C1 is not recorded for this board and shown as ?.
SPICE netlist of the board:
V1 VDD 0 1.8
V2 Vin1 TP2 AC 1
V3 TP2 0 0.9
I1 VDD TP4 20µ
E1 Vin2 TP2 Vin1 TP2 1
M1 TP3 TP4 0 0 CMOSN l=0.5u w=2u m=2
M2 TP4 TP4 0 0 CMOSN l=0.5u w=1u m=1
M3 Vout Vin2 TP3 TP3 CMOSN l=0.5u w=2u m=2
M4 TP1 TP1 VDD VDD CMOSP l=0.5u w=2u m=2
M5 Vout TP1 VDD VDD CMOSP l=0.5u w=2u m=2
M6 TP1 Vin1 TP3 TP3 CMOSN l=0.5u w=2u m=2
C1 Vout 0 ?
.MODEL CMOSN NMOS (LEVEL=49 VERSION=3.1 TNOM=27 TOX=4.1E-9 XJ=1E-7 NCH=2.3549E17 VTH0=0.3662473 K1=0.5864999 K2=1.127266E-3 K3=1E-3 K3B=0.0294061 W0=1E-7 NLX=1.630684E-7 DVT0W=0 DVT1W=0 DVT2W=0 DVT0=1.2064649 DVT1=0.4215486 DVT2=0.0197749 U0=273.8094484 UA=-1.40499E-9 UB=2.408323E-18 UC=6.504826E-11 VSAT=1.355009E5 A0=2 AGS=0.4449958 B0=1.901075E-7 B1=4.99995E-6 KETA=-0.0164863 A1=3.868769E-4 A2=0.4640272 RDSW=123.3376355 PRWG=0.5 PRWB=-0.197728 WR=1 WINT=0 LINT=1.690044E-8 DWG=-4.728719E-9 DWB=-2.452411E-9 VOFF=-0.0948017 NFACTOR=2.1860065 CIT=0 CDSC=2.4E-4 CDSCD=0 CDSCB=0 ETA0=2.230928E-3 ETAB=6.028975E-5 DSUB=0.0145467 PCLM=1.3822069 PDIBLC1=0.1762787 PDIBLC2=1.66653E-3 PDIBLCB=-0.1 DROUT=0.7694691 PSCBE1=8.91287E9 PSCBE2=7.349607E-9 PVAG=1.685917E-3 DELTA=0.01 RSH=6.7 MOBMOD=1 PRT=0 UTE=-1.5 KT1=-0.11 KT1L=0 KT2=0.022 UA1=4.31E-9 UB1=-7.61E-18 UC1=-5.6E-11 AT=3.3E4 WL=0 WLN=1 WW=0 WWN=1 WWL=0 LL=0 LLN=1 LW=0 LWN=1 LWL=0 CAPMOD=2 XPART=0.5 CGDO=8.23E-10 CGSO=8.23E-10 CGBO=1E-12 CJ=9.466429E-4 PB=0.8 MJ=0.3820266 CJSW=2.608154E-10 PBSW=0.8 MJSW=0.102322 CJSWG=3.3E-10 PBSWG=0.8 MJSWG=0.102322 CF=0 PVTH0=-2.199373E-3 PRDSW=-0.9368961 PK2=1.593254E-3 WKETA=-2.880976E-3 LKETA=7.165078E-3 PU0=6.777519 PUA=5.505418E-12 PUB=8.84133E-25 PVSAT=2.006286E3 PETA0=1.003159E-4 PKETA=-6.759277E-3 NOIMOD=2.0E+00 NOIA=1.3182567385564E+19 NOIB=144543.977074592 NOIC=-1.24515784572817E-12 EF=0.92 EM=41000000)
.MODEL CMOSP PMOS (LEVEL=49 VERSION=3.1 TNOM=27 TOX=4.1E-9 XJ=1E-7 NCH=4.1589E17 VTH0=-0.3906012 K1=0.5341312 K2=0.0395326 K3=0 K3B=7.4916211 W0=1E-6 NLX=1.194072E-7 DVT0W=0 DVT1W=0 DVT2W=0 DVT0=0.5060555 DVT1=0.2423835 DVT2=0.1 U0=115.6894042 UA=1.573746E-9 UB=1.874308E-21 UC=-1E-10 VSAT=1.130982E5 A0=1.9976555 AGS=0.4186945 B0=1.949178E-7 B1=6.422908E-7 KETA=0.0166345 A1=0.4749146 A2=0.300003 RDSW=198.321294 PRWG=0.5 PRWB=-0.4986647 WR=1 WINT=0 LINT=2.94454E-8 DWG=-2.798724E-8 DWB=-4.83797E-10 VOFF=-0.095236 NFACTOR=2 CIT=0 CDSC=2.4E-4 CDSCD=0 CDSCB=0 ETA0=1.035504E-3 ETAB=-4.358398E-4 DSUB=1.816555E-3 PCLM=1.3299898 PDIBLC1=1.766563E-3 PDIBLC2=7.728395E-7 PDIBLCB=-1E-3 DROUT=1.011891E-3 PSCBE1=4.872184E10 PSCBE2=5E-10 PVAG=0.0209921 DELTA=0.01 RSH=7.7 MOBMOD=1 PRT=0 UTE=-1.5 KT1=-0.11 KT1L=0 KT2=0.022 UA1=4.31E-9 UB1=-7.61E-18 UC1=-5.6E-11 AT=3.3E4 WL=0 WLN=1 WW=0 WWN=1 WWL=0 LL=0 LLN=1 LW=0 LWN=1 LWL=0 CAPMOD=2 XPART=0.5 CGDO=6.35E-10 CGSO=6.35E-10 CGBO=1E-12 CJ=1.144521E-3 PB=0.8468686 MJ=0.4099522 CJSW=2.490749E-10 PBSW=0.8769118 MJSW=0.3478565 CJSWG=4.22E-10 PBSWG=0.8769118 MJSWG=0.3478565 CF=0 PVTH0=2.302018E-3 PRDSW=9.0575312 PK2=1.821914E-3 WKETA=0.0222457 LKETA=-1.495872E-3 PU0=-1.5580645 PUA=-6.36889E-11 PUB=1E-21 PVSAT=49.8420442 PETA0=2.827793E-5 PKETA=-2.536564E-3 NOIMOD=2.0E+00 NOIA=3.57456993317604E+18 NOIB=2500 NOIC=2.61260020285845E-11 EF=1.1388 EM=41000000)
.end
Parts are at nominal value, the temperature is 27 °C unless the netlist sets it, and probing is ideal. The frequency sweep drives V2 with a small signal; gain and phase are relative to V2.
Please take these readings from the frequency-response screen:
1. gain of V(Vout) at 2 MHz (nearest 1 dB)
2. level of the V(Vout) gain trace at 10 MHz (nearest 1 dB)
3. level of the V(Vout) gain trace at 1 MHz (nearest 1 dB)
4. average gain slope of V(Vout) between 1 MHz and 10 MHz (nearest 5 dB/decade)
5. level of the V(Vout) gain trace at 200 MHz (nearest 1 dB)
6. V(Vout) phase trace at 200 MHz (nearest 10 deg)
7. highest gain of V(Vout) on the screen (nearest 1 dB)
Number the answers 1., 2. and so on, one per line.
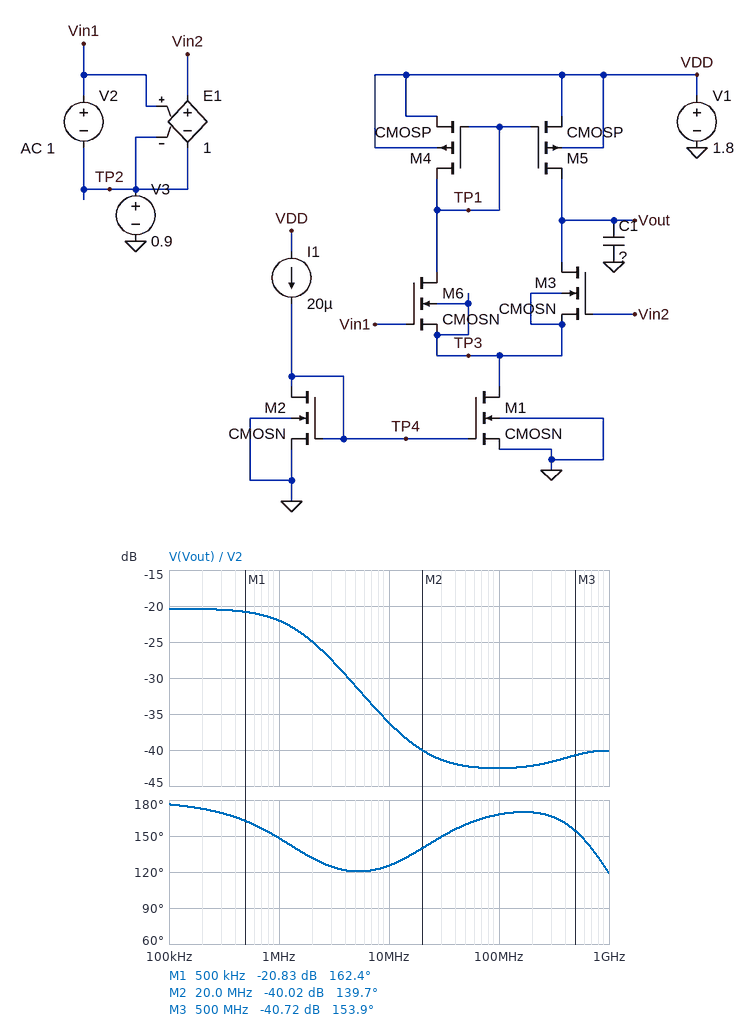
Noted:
1. -25 dB
2. -36 dB
3. -22 dB
4. -15 dB/decade
5. -42 dB
6. 170 deg
7. -20 dB
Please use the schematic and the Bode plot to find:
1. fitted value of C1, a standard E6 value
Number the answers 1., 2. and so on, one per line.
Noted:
1. 680 fF
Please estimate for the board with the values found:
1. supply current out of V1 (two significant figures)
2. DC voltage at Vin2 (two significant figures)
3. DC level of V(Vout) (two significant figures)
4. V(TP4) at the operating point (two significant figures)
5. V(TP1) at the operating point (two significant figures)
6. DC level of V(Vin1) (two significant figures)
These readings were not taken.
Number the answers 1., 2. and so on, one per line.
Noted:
1. 91 µA
2. 900 mV
3. 980 mV
4. 720 mV
5. 980 mV
6. 900 mV
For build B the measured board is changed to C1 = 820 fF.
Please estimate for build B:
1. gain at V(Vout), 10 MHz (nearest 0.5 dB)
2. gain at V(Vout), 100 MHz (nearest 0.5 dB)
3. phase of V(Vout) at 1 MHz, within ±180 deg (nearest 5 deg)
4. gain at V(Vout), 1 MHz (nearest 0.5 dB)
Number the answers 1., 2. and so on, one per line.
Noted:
1. -38.0 dB
2. -44.0 dB
3. 145 deg
4. -22.5 dB
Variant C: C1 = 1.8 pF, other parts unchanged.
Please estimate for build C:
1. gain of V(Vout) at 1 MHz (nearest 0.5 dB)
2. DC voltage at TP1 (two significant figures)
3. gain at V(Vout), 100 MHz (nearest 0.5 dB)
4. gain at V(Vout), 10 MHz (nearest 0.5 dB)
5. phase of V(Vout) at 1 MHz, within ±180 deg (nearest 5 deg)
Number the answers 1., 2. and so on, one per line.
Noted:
1. -26.5 dB
2. 980 mV
3. -51.0 dB
4. -44.5 dB
5. 120 deg
